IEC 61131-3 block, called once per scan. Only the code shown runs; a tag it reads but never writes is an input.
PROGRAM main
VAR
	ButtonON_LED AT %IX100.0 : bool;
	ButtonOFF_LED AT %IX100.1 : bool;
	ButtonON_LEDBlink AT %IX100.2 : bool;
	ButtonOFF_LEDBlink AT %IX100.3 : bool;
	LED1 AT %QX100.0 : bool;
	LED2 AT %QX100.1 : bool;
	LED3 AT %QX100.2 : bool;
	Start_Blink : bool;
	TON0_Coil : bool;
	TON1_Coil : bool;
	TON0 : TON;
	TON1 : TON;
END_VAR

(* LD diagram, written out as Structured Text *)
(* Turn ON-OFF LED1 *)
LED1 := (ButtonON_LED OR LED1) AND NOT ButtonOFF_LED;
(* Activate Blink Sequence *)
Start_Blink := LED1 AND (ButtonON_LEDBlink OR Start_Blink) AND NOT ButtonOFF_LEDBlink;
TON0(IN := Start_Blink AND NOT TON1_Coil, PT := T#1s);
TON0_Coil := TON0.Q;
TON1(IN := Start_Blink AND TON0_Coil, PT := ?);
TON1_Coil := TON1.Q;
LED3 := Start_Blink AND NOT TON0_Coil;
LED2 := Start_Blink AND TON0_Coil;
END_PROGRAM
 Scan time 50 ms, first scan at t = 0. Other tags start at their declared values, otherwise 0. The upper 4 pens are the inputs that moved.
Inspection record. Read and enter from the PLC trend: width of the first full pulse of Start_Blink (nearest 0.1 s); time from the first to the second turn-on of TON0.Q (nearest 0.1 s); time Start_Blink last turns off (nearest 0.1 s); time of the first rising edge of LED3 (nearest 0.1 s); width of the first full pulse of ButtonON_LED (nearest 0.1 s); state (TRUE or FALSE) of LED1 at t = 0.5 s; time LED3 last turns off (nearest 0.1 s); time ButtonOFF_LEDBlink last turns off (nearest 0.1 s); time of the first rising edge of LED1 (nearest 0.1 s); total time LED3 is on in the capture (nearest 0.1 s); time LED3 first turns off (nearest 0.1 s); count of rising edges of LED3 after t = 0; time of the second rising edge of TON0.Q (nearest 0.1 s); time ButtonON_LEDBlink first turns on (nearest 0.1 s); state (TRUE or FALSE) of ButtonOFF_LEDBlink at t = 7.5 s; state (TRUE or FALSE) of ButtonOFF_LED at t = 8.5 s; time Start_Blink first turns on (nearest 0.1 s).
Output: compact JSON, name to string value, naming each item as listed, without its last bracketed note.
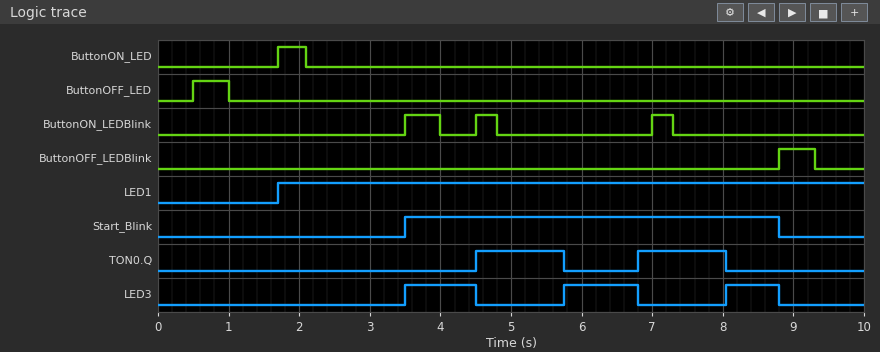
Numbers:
{"width of the first full pulse of Start_Blink": "5.3 s", "time from the first to the second turn-on of TON0.Q": "2.3 s", "time Start_Blink last turns off": "8.8 s", "time of the first rising edge of LED3": "3.5 s", "width of the first full pulse of ButtonON_LED": "0.4 s", "state (TRUE or FALSE) of LED1 at t = 0.5 s": "FALSE", "time LED3 last turns off": "8.8 s", "time ButtonOFF_LEDBlink last turns off": "9.3 s", "time of the first rising edge of LED1": "1.7 s", "total time LED3 is on in the capture": "2.8 s", "time LED3 first turns off": "4.5 s", "count of rising edges of LED3 after t = 0": "3", "time of the second rising edge of TON0.Q": "6.8 s", "time ButtonON_LEDBlink first turns on": "3.5 s", "state (TRUE or FALSE) of ButtonOFF_LEDBlink at t = 7.5 s": "FALSE", "state (TRUE or FALSE) of ButtonOFF_LED at t = 8.5 s": "FALSE", "time Start_Blink first turns on": "3.5 s"}
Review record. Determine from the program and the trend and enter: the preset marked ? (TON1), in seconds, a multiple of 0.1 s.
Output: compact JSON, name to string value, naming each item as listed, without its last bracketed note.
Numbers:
{"the preset marked ? (TON1), in seconds, a multiple of 0.1 s": "1.2 s"}
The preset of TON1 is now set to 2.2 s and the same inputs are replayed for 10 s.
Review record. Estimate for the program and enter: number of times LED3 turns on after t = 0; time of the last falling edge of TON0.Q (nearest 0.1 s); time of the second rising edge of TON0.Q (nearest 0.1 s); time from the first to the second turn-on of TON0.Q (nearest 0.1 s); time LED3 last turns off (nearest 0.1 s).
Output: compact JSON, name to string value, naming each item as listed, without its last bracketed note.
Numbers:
{"number of times LED3 turns on after t = 0": "2", "time of the last falling edge of TON0.Q": "8.8 s", "time of the second rising edge of TON0.Q": "7.8 s", "time from the first to the second turn-on of TON0.Q": "3.3 s", "time LED3 last turns off": "7.8 s"}
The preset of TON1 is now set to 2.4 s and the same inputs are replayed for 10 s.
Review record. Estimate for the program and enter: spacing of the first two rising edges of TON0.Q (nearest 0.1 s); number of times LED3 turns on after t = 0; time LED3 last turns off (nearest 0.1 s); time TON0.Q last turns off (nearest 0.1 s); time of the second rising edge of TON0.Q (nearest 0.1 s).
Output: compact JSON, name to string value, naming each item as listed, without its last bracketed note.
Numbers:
{"spacing of the first two rising edges of TON0.Q": "3.5 s", "number of times LED3 turns on after t = 0": "2", "time LED3 last turns off": "8.0 s", "time TON0.Q last turns off": "8.8 s", "time of the second rising edge of TON0.Q": "8.0 s"}
